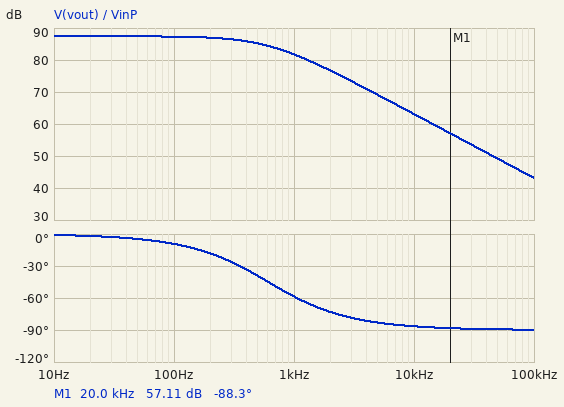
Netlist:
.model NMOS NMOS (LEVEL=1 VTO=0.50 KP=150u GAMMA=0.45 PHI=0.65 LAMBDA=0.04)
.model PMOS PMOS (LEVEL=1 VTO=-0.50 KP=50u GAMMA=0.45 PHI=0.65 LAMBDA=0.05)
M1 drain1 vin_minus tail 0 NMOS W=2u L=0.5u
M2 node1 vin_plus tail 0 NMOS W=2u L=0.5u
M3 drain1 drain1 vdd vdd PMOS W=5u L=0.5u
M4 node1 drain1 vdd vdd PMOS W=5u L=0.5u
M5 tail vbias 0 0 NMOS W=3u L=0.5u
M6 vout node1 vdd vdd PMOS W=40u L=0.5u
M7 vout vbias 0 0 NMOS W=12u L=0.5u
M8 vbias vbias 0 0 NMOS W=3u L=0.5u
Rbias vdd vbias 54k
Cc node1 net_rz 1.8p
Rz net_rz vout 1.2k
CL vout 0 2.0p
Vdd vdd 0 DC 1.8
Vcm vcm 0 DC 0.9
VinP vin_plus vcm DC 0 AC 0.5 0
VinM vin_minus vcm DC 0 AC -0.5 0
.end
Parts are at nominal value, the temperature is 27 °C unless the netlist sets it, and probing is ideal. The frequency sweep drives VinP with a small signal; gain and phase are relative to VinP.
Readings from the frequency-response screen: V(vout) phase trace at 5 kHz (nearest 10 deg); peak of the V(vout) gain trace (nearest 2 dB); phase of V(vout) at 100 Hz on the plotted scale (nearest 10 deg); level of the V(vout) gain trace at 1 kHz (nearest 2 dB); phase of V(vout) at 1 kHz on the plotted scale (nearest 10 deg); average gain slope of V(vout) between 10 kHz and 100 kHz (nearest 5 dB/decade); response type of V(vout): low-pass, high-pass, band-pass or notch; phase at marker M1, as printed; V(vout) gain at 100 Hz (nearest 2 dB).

-80 deg
88 dB
-10 deg
82 dB
-60 deg
-20 dB/decade
low-pass
-88.3 deg
88 dB
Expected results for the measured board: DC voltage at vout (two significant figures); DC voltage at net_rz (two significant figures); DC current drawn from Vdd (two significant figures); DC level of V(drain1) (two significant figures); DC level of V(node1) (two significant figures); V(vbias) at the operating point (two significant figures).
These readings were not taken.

420 mV
420 mV
120 µA
1.1 V
1.1 V
710 mV
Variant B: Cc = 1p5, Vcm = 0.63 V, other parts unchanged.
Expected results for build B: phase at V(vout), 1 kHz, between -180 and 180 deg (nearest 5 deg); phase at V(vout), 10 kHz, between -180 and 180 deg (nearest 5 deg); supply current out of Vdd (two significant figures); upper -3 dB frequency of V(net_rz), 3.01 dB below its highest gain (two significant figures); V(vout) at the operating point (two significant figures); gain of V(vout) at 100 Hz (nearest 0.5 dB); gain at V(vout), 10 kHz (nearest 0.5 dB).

-5 deg
-35 deg
48 µA
14 kHz
32 mV
48.5 dB
46.5 dB
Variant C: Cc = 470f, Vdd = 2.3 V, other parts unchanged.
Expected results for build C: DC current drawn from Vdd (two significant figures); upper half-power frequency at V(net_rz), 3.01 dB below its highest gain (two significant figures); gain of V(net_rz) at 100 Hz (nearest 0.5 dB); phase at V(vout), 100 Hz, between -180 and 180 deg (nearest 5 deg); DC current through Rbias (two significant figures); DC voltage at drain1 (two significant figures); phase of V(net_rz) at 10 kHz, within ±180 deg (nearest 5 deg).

160 µA
72 kHz
57.0 dB
0 deg
29 µA
1.6 V
-10 deg
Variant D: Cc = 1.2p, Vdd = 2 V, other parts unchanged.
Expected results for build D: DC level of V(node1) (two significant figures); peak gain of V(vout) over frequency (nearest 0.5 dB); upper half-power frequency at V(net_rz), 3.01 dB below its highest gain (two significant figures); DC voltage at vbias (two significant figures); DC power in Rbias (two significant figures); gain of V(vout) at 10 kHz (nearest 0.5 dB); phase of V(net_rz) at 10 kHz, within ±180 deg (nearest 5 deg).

1.3 V
64.0 dB
13 kHz
730 mV
30 µW
62.0 dB
-40 deg
